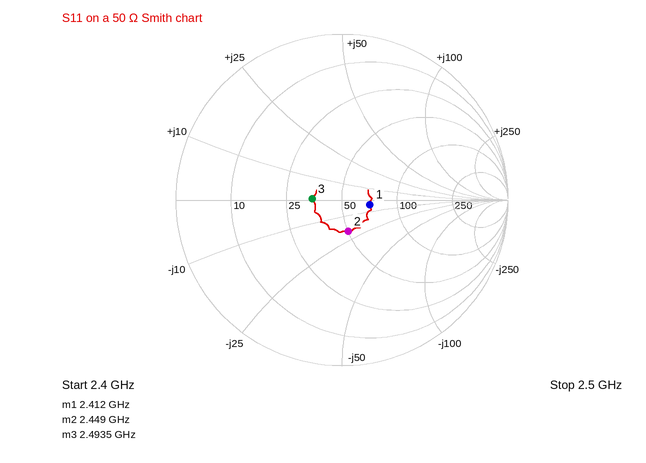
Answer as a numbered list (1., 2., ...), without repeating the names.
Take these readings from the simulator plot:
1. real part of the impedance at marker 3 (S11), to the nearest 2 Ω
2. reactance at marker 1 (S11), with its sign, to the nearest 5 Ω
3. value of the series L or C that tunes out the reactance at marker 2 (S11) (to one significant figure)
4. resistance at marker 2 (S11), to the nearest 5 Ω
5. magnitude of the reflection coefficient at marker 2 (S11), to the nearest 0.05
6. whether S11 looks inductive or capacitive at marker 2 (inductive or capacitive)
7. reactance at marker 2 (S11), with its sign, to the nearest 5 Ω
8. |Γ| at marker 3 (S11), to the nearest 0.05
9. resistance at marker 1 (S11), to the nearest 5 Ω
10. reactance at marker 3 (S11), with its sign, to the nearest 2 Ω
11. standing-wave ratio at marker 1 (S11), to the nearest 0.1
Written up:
1. 34 Ω
2. -5 Ω
3. 1 nH
4. 50 Ω
5. 0.20
6. capacitive
7. -20 Ω
8. 0.20
9. 70 Ω
10. 0 Ω
11. 1.4
